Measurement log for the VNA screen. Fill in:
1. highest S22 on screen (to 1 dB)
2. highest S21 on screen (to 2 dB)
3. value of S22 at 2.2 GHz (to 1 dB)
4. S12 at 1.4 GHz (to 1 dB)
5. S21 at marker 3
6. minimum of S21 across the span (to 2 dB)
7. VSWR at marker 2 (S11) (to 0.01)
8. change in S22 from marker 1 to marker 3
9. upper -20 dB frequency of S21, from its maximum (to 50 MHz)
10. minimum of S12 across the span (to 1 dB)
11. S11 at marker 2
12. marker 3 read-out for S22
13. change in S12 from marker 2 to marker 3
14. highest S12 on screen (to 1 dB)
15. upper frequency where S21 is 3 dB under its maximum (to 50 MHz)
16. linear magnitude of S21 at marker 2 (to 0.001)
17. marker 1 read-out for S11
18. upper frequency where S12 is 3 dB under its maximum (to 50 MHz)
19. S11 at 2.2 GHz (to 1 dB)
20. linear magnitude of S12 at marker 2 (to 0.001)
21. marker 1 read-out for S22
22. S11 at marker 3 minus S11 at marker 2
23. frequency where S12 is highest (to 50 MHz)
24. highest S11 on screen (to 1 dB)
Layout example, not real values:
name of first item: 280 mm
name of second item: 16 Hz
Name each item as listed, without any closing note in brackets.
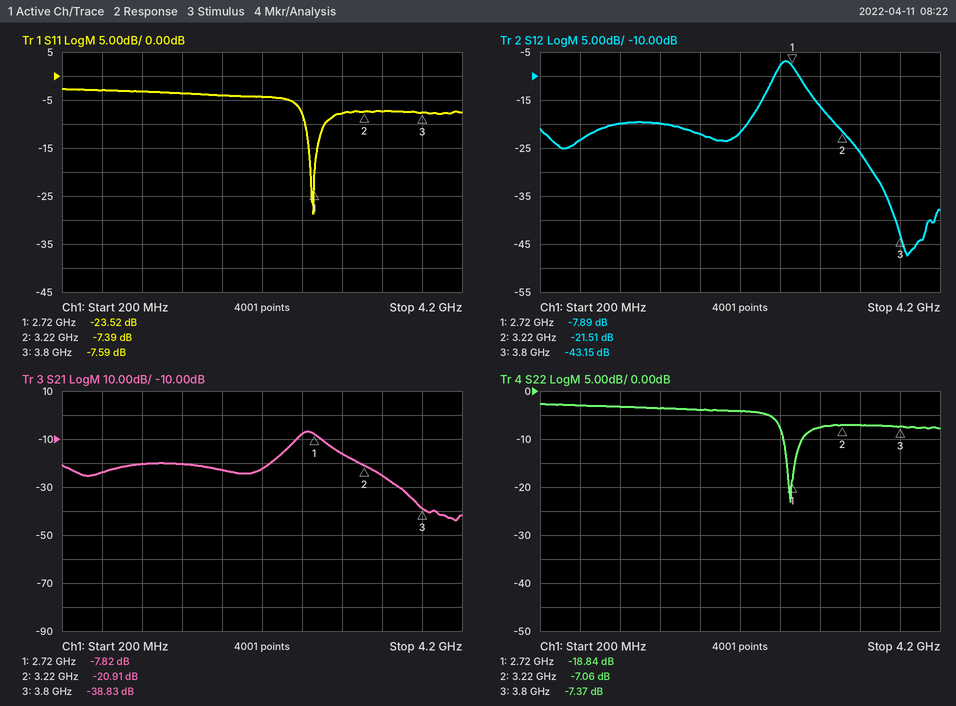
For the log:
highest S22 on screen: -3 dB
highest S21 on screen: -6 dB
value of S22 at 2.2 GHz: -4 dB
S12 at 1.4 GHz: -20 dB
S21 at marker 3: -38.83 dB
minimum of S21 across the span: -44 dB
VSWR at marker 2 (S11): 2.49
change in S22 from marker 1 to marker 3: 11.47 dB
upper -20 dB frequency of S21, from its maximum: 3.45 GHz
minimum of S12 across the span: -47 dB
S11 at marker 2: -7.39 dB
marker 3 read-out for S22: -7.37 dB
change in S12 from marker 2 to marker 3: -21.64 dB
highest S12 on screen: -7 dB
upper frequency where S21 is 3 dB under its maximum: 2.80 GHz
linear magnitude of S21 at marker 2: 0.090
marker 1 read-out for S11: -23.52 dB
upper frequency where S12 is 3 dB under its maximum: 2.80 GHz
S11 at 2.2 GHz: -4 dB
linear magnitude of S12 at marker 2: 0.084
marker 1 read-out for S22: -18.84 dB
S11 at marker 3 minus S11 at marker 2: -0.20 dB
frequency where S12 is highest: 2.65 GHz
highest S11 on screen: -3 dB
